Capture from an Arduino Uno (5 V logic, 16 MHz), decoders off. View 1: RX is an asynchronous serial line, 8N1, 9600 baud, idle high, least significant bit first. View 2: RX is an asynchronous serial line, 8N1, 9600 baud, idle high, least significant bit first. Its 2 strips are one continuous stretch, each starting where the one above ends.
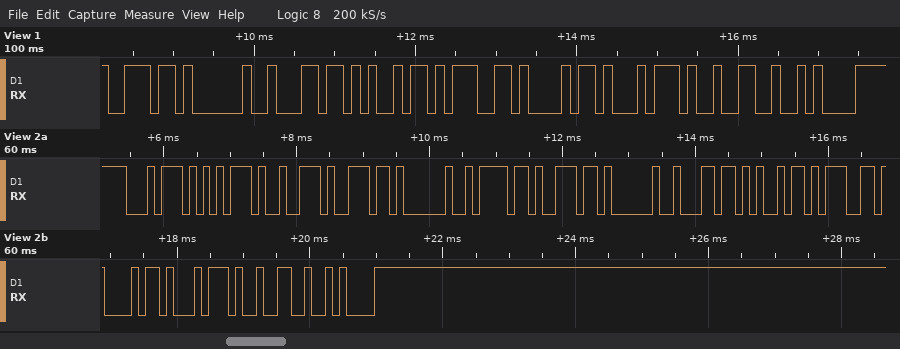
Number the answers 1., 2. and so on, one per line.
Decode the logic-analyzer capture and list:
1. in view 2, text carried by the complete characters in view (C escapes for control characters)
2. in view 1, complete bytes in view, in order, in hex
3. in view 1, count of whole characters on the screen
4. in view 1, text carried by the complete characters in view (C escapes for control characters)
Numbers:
1. "turn on light2\n"
2. 6E 20 6C 69 67 68 74 32 0A
3. 9
4. "n light2\n"
